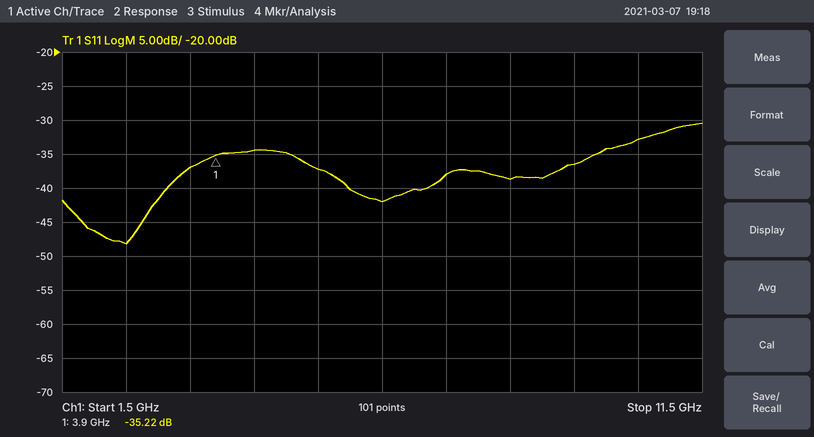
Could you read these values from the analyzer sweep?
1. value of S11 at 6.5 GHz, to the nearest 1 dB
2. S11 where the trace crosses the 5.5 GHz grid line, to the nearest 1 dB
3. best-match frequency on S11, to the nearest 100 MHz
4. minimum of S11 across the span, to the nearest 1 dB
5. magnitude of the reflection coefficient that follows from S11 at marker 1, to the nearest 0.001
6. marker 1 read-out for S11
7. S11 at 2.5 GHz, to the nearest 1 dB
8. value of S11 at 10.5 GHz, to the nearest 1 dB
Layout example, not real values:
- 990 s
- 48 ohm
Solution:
- -42 dB
- -37 dB
- 2.5 GHz
- -48 dB
- 0.017
- -35.22 dB
- -48 dB
- -33 dB
